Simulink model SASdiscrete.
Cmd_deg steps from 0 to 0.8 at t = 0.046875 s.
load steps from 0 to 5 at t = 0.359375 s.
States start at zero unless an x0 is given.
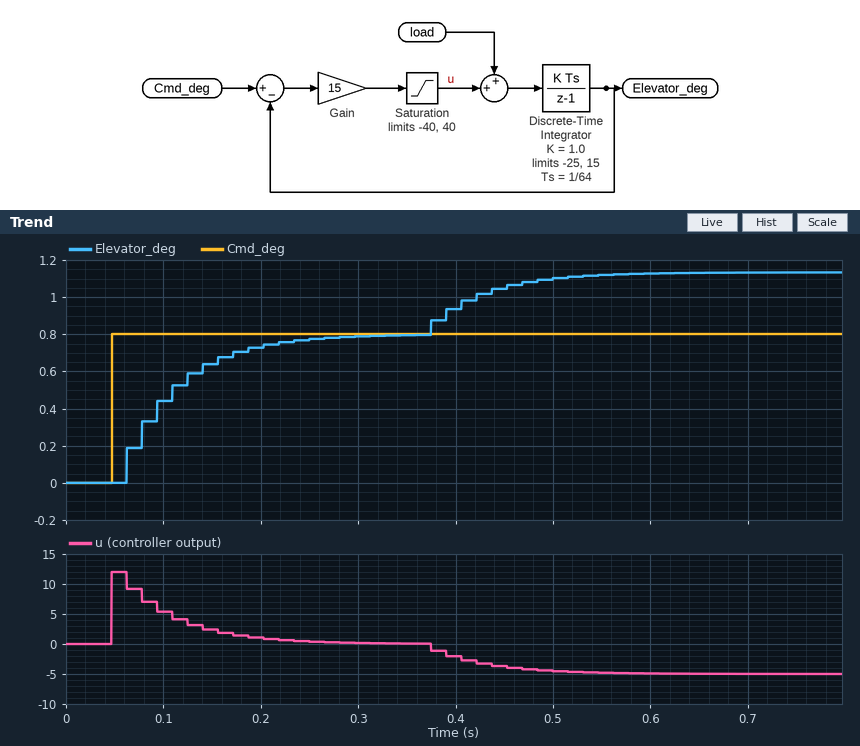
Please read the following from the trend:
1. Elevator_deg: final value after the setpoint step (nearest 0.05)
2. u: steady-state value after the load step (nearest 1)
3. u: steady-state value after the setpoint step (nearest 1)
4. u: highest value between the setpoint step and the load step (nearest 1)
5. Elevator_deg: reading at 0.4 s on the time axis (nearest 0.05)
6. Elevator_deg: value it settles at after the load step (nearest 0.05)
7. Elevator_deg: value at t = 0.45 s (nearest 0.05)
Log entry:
0.80
-5
0
12
0.95
1.15
1.05
